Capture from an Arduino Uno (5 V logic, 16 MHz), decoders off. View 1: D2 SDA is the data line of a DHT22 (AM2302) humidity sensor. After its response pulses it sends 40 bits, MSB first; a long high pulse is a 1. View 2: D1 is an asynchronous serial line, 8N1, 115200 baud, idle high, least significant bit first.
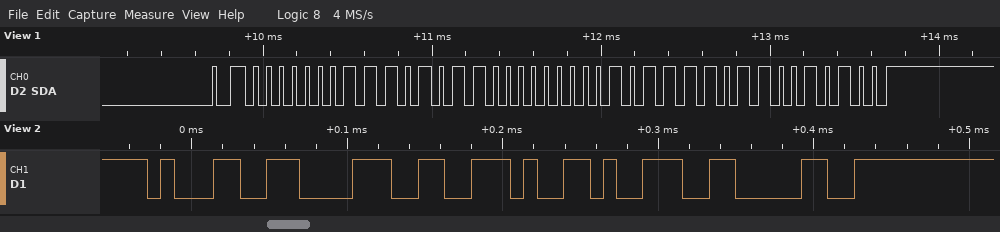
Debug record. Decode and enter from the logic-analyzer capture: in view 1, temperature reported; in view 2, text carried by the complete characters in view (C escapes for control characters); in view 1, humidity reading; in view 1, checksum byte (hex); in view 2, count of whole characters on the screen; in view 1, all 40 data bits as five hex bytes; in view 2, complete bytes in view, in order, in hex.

18.9 °C
"18.90"
47.0 %
0x94
5
01 D6 00 BD 94
0x31 0x38 0x2E 0x39 0x30
